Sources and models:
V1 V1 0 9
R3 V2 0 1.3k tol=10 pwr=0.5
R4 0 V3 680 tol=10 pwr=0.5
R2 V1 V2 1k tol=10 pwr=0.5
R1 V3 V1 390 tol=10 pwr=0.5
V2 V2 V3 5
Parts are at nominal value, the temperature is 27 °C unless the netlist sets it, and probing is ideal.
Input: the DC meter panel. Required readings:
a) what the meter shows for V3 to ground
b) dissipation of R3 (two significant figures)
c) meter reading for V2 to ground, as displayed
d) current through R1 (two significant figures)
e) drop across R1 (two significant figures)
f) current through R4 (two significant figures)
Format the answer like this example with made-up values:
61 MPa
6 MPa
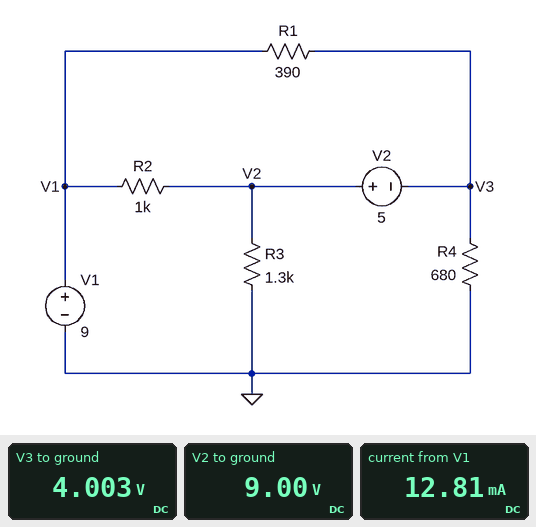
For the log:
4.003 V
62 mW
9.00 V
13 mA
5.0 V
5.9 mA
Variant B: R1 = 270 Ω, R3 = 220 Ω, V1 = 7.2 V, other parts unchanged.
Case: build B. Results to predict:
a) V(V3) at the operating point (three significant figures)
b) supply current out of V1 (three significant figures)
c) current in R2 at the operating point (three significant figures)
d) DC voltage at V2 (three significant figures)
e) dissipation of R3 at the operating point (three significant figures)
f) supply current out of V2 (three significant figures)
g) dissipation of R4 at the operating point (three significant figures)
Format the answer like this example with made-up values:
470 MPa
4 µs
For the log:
573 mV
26.2 mA
1.63 mA
5.57 V
141 mW
23.7 mA
482 µW
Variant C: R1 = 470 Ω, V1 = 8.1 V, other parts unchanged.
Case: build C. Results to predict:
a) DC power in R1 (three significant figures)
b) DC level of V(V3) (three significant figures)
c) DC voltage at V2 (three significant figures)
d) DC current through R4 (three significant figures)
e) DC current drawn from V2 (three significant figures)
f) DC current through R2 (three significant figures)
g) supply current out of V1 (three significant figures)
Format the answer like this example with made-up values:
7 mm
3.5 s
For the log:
53.8 mW
3.07 V
8.07 V
4.52 mA
6.18 mA
28.2 µA
10.7 mA
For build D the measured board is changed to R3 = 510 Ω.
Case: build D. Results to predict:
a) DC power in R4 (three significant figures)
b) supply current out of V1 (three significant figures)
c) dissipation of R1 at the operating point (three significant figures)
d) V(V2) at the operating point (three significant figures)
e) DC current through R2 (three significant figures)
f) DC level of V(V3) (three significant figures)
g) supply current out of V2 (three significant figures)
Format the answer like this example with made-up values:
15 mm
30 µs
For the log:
8.97 mW
18.3 mA
109 mW
7.47 V
1.53 mA
2.47 V
13.1 mA
